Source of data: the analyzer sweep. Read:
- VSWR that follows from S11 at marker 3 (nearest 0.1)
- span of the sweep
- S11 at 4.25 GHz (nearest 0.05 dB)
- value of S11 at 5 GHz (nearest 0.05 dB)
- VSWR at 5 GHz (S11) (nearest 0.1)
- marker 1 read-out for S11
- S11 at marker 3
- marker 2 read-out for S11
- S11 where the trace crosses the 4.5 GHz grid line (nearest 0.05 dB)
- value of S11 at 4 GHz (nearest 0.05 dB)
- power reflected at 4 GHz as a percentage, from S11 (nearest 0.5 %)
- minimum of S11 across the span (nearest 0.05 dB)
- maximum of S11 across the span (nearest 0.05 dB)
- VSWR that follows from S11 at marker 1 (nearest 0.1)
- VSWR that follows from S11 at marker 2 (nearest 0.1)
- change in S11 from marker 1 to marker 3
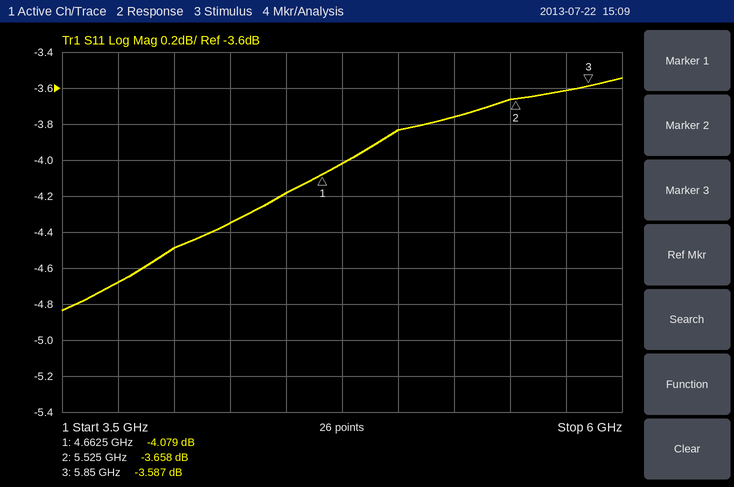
4.9
2.5 GHz
-4.35 dB
-3.85 dB
4.6
-4.079 dB
-3.587 dB
-3.658 dB
-4.20 dB
-4.50 dB
35.5 %
-4.85 dB
-3.55 dB
4.3
4.8
0.492 dB
